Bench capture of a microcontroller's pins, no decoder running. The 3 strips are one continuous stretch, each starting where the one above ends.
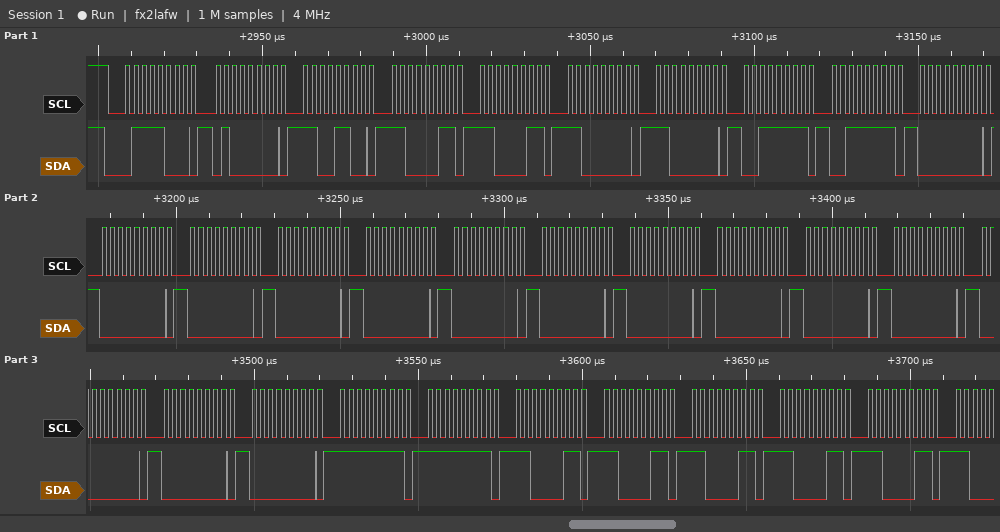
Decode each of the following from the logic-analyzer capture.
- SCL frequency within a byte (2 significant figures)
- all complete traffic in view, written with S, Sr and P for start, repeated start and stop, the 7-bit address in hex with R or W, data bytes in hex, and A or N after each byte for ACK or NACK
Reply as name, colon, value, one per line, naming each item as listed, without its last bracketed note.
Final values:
SCL frequency within a byte: 400 kHz
all complete traffic in view, written with S, Sr and P for start, repeated start and stop, the 7-bit address in hex with R or W, data bytes in hex, and A or N after each byte for ACK or NACK: S 3CW A 40 A CC A C3 A C3 A C0 A C0 A 3F A 3F A 00 A 00 A 00 A 00 A 00 A 00 A 00 A 00 A 00 A 00 A 00 A 00 A 00 A 00 A FF A FF A C3 A C3 A C3 A C3 A C3 A
